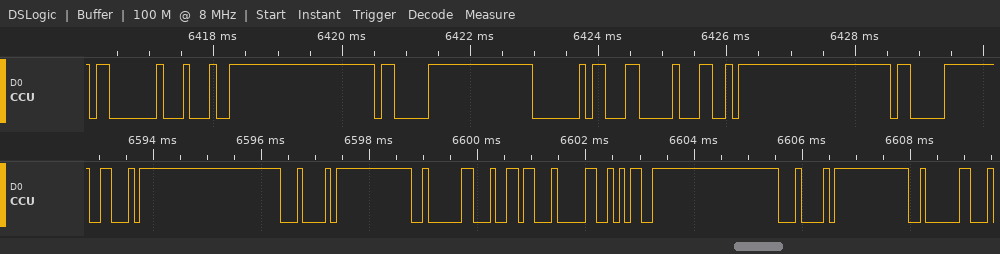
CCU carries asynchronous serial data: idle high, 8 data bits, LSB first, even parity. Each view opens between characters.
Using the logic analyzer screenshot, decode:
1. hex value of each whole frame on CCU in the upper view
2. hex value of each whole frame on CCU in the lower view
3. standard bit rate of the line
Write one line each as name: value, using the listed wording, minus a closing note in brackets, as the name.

hex value of each whole frame on CCU in the upper view: 03, 44, 83, 40, 0C, 4C, 83
hex value of each whole frame on CCU in the lower view: 46, 84, 02, 64, 04, 6A, 84, 02
standard bit rate of the line: 9600 baud
